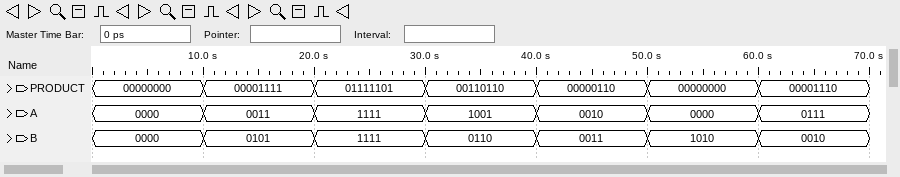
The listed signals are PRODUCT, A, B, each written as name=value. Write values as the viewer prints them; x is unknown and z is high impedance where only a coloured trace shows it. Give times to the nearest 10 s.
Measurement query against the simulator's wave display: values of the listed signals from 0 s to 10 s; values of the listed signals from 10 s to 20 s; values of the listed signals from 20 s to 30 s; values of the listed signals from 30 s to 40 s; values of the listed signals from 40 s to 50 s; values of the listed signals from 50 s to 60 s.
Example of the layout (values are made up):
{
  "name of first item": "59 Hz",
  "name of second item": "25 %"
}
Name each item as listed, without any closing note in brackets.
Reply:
{
  "values of the listed signals from 0 s to 10 s": "PRODUCT=00000000, A=0000, B=0000",
  "values of the listed signals from 10 s to 20 s": "PRODUCT=00001111, A=0011, B=0101",
  "values of the listed signals from 20 s to 30 s": "PRODUCT=01111101, A=1111, B=1111",
  "values of the listed signals from 30 s to 40 s": "PRODUCT=00110110, A=1001, B=0110",
  "values of the listed signals from 40 s to 50 s": "PRODUCT=00000110, A=0010, B=0011",
  "values of the listed signals from 50 s to 60 s": "PRODUCT=00000000, A=0000, B=1010"
}
